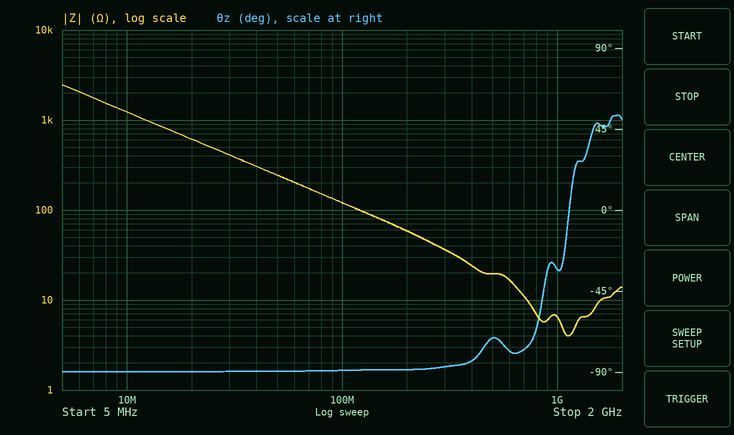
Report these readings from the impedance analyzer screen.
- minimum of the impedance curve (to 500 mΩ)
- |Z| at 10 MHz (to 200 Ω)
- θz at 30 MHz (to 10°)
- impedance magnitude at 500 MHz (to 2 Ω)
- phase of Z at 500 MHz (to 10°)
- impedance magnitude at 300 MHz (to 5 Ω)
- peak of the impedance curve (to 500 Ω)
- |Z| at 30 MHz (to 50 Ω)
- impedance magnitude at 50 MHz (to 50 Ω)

4.0 Ω
1.2 kΩ
-90°
20 Ω
-70°
35 Ω
2.5 kΩ
400 Ω
250 Ω
